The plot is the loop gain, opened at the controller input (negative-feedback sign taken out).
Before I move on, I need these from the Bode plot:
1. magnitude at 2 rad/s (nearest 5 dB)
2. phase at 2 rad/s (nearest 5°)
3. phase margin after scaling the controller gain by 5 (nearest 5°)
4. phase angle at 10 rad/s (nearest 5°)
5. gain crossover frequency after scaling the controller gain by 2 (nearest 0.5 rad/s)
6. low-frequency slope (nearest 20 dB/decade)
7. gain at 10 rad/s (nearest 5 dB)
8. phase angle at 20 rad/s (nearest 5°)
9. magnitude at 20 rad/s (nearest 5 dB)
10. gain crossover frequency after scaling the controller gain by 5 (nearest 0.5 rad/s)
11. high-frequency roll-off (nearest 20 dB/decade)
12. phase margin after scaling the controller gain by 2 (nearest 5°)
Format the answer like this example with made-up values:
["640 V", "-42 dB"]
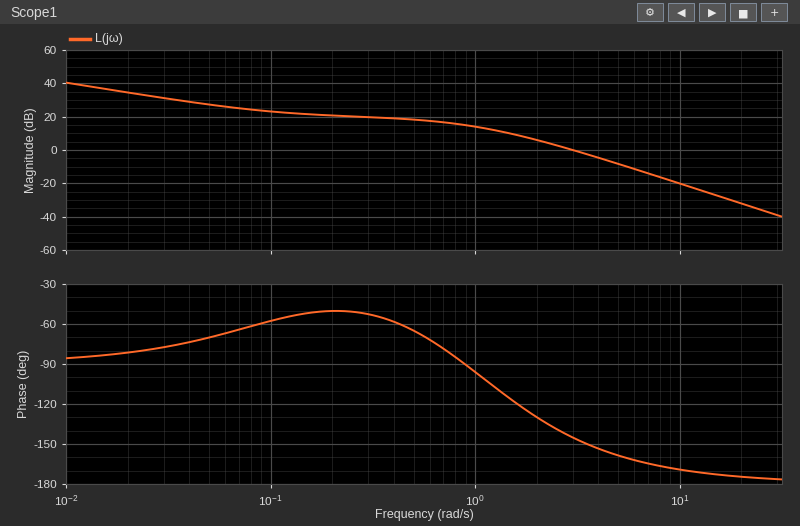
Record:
["5 dB", "-130°", "15°", "-170°", "4.5 rad/s", "-20 dB/decade", "-20 dB", "-175°", "-30 dB", "7.0 rad/s", "-40 dB/decade", "25°"]
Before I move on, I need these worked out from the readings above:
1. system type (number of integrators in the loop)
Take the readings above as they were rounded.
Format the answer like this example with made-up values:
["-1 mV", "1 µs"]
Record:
["1"]
